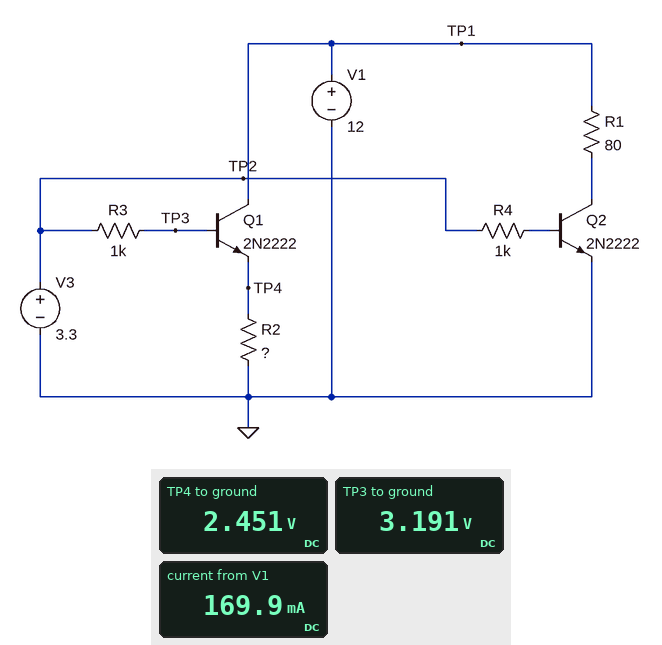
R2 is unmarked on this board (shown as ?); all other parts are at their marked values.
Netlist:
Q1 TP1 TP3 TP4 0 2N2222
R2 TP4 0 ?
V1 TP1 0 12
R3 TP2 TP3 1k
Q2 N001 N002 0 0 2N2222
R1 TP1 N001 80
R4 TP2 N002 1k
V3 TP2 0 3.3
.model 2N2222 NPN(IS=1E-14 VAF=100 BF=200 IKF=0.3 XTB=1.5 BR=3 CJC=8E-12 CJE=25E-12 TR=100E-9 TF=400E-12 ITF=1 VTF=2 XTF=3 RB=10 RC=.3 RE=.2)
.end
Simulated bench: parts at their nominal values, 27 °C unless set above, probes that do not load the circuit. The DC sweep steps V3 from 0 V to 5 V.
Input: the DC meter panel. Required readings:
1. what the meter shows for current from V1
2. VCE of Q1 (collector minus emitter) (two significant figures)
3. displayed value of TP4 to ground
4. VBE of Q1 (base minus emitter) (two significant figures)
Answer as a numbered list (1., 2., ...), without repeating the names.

1. 169.9 mA
2. 9.5 V
3. 2.451 V
4. 740 mV
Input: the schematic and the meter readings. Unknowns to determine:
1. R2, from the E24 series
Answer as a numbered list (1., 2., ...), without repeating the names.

1. 110 Ω
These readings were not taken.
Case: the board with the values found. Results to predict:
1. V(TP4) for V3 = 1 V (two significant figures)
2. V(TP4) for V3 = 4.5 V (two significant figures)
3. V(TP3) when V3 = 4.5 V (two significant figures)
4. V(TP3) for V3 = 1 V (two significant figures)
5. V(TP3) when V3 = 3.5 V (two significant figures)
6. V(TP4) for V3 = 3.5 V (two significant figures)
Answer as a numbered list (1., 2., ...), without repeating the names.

1. 310 mV
2. 3.6 V
3. 4.3 V
4. 990 mV
5. 3.4 V
6. 2.6 V
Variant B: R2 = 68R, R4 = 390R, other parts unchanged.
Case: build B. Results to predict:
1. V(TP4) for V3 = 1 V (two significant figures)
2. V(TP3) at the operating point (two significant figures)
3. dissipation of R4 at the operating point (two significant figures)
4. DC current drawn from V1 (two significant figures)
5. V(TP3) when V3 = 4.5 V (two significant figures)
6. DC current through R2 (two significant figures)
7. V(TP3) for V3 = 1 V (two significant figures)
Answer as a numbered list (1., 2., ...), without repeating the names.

1. 290 mV
2. 3.1 V
3. 15 mW
4. 180 mA
5. 4.2 V
6. 35 mA
7. 980 mV
